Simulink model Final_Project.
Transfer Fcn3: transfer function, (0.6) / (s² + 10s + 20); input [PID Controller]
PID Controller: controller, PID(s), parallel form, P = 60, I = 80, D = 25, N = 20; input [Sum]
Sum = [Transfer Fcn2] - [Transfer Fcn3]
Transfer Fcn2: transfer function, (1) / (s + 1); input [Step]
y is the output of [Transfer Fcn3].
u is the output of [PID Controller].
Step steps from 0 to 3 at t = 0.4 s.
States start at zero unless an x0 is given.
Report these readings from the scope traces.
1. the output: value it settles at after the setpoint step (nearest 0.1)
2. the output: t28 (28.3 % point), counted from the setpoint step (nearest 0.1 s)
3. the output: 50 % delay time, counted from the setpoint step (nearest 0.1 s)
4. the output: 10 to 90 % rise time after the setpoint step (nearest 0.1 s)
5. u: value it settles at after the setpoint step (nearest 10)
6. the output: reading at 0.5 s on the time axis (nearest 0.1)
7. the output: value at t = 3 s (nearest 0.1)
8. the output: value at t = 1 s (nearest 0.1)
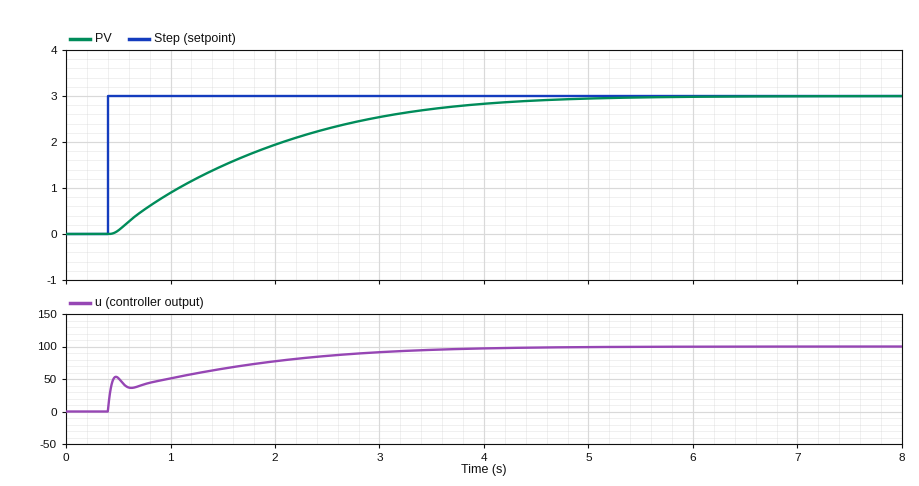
3.0
0.6 s
1.1 s
2.8 s
100
0.1
2.5
0.9
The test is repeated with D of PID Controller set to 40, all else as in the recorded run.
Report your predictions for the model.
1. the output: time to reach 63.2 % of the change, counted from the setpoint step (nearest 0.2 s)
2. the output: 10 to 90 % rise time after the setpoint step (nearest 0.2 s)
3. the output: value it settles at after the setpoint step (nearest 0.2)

1.6 s
3.0 s
3.0
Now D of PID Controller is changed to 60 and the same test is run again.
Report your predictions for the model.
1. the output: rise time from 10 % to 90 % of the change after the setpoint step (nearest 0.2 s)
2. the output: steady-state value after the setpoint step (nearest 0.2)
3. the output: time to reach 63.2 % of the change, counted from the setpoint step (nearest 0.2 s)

3.2 s
3.0
1.6 s
